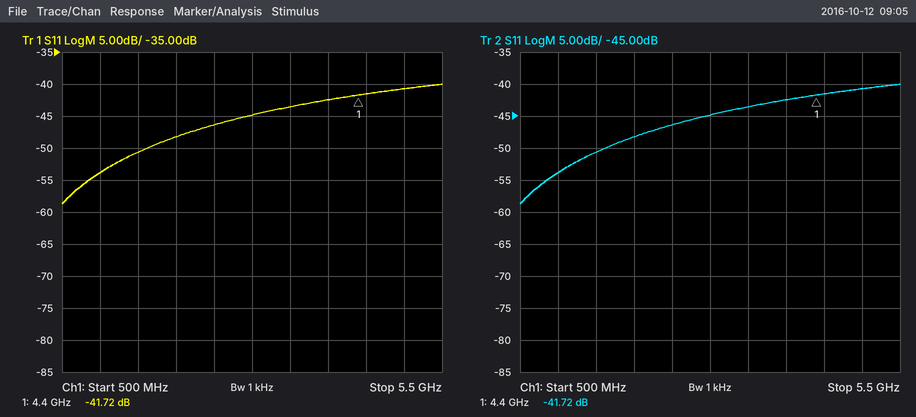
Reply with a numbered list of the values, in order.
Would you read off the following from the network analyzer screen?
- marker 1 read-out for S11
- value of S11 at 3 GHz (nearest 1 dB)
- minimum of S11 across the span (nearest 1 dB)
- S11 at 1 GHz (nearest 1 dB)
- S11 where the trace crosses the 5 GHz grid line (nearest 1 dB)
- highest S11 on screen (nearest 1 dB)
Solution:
1. -41.72 dB
2. -45 dB
3. -59 dB
4. -54 dB
5. -41 dB
6. -40 dB
